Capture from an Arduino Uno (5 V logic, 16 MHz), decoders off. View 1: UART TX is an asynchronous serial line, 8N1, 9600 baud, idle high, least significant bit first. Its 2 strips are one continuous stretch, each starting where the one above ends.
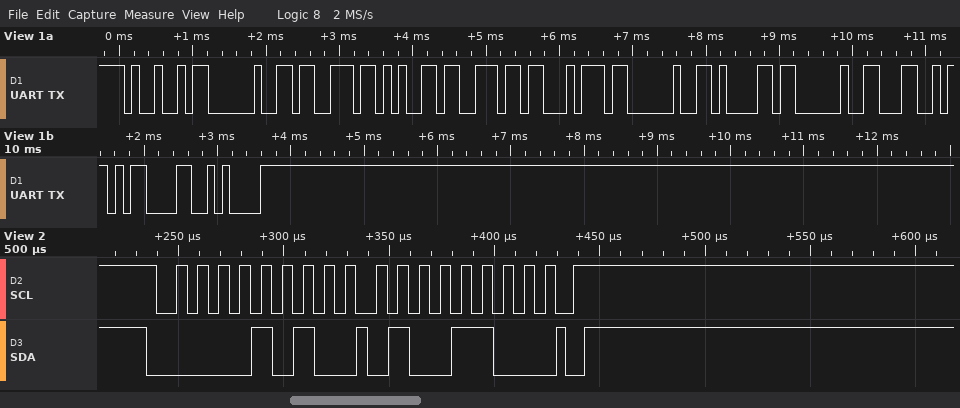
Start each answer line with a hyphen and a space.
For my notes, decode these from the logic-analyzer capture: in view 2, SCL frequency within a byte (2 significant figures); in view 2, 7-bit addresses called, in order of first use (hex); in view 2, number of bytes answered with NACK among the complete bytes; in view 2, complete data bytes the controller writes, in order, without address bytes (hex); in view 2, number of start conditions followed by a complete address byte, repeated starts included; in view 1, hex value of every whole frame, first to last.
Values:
- 100 kHz
- 0x05
- 0
- 4C
- 1
- 49 20 73 65 6E 74 20 61 20 4C 0D 0A
